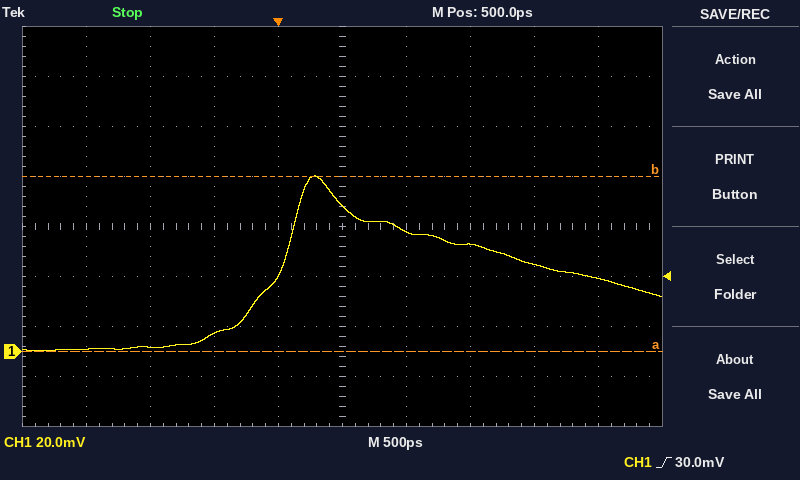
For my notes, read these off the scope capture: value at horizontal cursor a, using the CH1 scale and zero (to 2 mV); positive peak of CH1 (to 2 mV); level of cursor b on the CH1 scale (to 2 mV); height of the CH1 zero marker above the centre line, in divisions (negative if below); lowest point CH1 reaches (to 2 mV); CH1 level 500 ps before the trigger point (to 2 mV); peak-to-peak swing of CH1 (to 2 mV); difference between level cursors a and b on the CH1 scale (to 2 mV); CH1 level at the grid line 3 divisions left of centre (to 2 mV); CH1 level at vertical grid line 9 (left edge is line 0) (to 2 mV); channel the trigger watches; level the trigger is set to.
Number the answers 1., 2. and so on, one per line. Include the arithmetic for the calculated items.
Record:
1. 0 mV
2. 70 mV
3. 70 mV
4. -2.5 div
5. 0 mV
6. 8 mV
7. 70 mV − (0 mV) = 70 mV
8. 70 mV
9. 2 mV
10. 30 mV
11. CH1
12. 30.0 mV
